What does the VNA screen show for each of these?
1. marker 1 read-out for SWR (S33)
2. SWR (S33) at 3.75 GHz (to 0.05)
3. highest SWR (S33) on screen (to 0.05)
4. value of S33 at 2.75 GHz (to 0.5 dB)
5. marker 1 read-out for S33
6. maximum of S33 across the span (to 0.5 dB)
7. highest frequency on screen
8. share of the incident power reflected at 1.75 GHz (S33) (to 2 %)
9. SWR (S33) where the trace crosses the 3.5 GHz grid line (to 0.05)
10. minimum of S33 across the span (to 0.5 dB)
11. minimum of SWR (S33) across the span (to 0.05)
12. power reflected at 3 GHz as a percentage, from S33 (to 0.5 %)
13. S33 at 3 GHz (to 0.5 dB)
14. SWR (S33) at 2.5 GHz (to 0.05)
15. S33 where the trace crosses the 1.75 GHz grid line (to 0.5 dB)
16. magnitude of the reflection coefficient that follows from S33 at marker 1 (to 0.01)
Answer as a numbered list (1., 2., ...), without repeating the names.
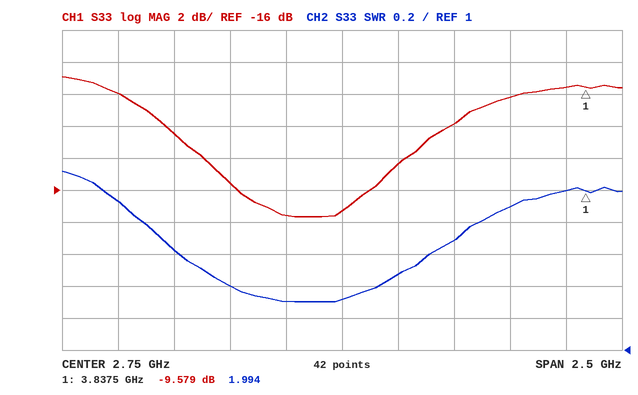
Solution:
1. 1.994
2. 2.00
3. 2.10
4. -17.5 dB
5. -9.579 dB
6. -9.0 dB
7. 4 GHz
8. 10 %
9. 1.90
10. -17.5 dB
11. 1.30
12. 3.5 %
13. -14.5 dB
14. 1.30
15. -10.0 dB
16. 0.33
